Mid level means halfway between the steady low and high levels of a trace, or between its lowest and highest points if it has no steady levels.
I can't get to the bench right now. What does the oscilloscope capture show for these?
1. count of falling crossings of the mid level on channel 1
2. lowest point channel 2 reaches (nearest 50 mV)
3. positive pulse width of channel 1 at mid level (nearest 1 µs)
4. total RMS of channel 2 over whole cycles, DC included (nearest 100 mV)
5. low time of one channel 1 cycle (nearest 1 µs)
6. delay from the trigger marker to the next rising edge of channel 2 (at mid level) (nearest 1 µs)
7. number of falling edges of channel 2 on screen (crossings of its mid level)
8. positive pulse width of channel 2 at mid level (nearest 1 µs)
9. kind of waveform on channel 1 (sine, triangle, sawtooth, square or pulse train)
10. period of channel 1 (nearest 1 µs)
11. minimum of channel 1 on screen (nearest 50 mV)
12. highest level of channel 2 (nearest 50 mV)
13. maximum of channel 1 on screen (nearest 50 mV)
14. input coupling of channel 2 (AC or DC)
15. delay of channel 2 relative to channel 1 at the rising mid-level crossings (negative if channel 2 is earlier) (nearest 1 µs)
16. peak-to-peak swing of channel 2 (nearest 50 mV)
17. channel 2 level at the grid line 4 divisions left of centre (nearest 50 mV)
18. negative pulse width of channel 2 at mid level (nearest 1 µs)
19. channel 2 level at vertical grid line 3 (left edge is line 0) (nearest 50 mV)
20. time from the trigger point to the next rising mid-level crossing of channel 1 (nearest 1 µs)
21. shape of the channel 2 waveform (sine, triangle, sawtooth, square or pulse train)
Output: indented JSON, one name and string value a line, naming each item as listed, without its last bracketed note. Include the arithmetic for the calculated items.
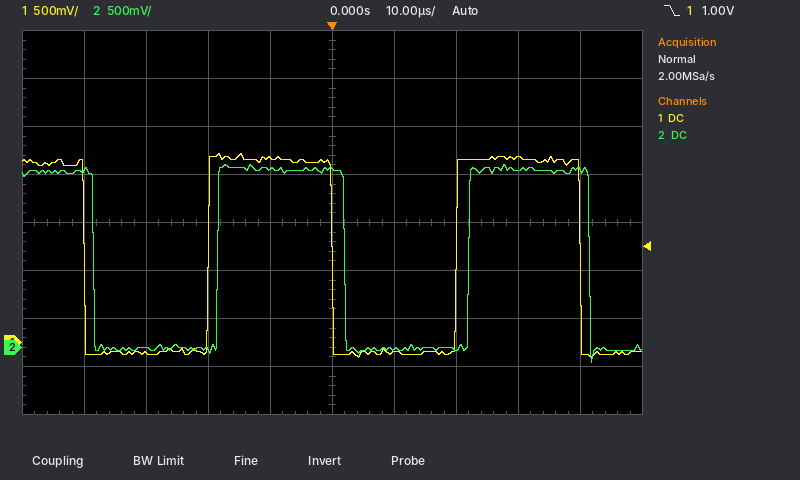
{
  "count of falling crossings of the mid level on channel 1": "3",
  "lowest point channel 2 reaches": "-150 mV",
  "positive pulse width of channel 1 at mid level": "20 µs",
  "total RMS of channel 2 over whole cycles, DC included": "√(0.5 × (1.90 V)² + 0.5 × (-150 mV)²) ≈ 1.3 V",
  "low time of one channel 1 cycle": "20 µs",
  "delay from the trigger marker to the next rising edge of channel 2 (at mid level)": "22 µs",
  "number of falling edges of channel 2 on screen": "3",
  "positive pulse width of channel 2 at mid level": "20 µs",
  "kind of waveform on channel 1": "square",
  "period of channel 1": "40 µs",
  "minimum of channel 1 on screen": "-150 mV",
  "highest level of channel 2": "1.90 V",
  "maximum of channel 1 on screen": "1.95 V",
  "input coupling of channel 2": "DC",
  "delay of channel 2 relative to channel 1 at the rising mid-level crossings (negative if channel 2 is earlier)": "+2 µs",
  "peak-to-peak swing of channel 2": "1.90 V − (-150 mV) = 2.05 V",
  "channel 2 level at the grid line 4 divisions left of centre": "1.85 V",
  "negative pulse width of channel 2 at mid level": "20 µs",
  "channel 2 level at vertical grid line 3 (left edge is line 0)": "-50 mV",
  "time from the trigger point to the next rising mid-level crossing of channel 1": "20 µs",
  "shape of the channel 2 waveform": "square"
}
